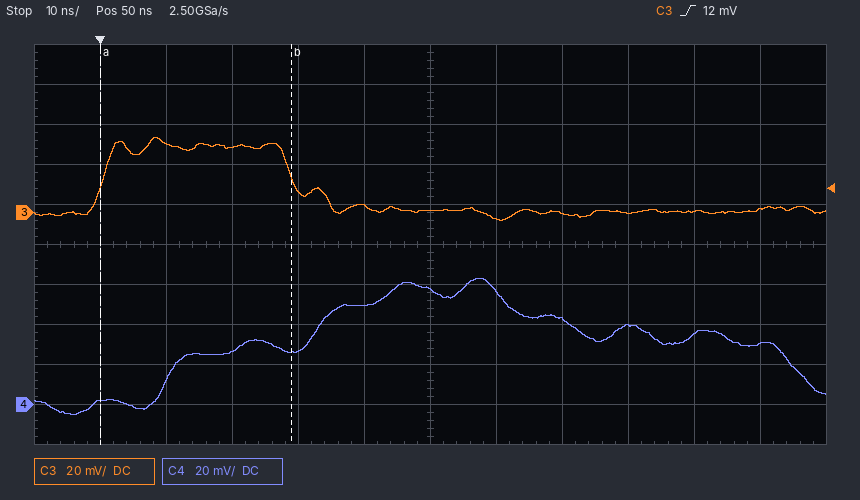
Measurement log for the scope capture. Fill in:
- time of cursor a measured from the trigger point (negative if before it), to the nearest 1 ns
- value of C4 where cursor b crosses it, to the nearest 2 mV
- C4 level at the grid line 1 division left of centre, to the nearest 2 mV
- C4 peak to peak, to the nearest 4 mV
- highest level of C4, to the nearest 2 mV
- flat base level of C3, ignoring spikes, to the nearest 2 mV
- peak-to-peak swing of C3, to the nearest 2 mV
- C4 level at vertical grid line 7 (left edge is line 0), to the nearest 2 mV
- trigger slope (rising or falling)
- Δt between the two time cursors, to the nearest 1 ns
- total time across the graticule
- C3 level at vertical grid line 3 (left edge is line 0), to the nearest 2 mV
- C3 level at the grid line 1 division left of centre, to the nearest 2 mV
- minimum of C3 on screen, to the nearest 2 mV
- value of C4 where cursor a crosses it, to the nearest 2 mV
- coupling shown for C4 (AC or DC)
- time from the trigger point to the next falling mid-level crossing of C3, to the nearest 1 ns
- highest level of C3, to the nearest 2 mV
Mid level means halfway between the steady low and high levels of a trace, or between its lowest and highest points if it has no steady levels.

0 ns
26 mV
50 mV
68 mV
64 mV
0 mV
42 mV
56 mV
rising
29 ns
120 ns
32 mV
4 mV
-4 mV
2 mV
DC
29 ns
38 mV
